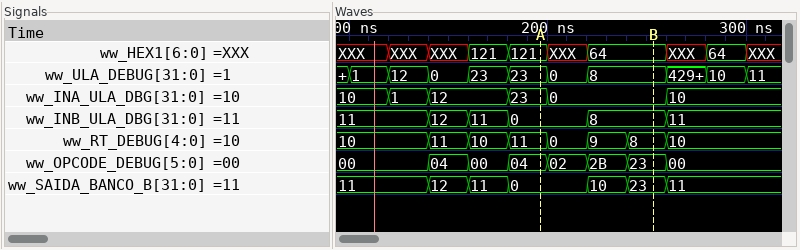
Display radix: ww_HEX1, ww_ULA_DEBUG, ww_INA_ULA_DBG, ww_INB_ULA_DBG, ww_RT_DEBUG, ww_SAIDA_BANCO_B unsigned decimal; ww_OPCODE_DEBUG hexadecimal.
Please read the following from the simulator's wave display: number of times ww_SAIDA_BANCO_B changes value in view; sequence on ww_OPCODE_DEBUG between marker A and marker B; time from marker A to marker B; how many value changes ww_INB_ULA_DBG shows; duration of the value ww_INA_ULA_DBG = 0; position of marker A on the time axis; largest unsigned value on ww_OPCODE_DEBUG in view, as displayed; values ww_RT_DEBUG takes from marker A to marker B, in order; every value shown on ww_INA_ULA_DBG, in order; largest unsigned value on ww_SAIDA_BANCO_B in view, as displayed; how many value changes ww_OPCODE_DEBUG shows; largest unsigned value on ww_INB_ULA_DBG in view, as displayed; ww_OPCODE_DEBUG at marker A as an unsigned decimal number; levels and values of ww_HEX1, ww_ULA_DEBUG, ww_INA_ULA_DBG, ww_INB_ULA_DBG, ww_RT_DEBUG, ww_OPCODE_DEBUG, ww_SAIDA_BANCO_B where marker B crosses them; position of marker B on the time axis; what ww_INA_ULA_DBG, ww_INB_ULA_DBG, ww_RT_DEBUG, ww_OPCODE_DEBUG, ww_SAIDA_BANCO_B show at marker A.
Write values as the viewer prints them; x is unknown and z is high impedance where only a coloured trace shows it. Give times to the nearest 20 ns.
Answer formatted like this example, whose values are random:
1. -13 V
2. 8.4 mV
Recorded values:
1. 6
2. 04, 02, 2B, 23
3. 60 ns
4. 5
5. 60 ns
6. 200 ns
7. 2B
8. 11, 0, 9, 8
9. 10, 1, 12, 23, 0, 10
10. 23
11. 7
12. 12
13. 4
14. ww_HEX1=64, ww_ULA_DEBUG=8, ww_INA_ULA_DBG=0, ww_INB_ULA_DBG=8, ww_RT_DEBUG=8, ww_OPCODE_DEBUG=23, ww_SAIDA_BANCO_B=23
15. 260 ns
16. ww_INA_ULA_DBG=23, ww_INB_ULA_DBG=0, ww_RT_DEBUG=11, ww_OPCODE_DEBUG=04, ww_SAIDA_BANCO_B=0
